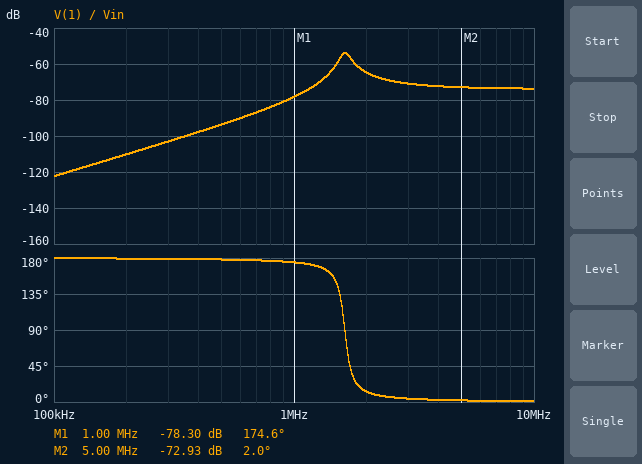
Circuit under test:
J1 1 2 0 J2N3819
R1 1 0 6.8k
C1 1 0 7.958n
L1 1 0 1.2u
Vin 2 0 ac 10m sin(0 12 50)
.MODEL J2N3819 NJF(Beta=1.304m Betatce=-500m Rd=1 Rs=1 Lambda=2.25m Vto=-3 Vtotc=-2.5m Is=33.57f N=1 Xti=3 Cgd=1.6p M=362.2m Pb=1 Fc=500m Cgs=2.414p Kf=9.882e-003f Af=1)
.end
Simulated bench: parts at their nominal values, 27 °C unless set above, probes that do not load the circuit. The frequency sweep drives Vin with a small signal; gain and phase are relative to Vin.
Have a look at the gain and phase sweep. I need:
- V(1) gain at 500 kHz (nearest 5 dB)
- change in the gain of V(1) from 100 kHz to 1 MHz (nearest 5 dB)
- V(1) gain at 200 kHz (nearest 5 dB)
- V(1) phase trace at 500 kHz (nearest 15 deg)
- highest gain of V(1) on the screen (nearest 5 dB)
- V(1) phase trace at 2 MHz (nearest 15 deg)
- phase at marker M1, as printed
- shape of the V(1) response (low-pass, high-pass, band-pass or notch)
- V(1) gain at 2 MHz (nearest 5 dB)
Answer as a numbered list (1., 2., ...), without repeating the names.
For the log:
1. -95 dB
2. 45 dB
3. -110 dB
4. 180 deg
5. -55 dB
6. 15 deg
7. 174.6 deg
8. high-pass
9. -65 dB
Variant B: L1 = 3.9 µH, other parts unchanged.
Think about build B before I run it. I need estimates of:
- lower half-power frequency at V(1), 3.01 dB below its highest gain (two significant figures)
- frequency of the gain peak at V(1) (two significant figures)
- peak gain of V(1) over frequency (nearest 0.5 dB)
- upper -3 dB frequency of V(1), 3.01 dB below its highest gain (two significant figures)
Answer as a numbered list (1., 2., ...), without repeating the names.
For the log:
1. 840 kHz
2. 910 kHz
3. -58.5 dB
4. 1.0 MHz
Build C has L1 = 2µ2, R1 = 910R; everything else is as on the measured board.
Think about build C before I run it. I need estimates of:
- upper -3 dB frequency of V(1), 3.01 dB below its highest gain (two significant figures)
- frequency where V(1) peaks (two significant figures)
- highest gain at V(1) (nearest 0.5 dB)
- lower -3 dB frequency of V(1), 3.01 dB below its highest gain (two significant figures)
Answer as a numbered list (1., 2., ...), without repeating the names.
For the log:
1. 1.3 MHz
2. 1.2 MHz
3. -57.0 dB
4. 1.1 MHz
